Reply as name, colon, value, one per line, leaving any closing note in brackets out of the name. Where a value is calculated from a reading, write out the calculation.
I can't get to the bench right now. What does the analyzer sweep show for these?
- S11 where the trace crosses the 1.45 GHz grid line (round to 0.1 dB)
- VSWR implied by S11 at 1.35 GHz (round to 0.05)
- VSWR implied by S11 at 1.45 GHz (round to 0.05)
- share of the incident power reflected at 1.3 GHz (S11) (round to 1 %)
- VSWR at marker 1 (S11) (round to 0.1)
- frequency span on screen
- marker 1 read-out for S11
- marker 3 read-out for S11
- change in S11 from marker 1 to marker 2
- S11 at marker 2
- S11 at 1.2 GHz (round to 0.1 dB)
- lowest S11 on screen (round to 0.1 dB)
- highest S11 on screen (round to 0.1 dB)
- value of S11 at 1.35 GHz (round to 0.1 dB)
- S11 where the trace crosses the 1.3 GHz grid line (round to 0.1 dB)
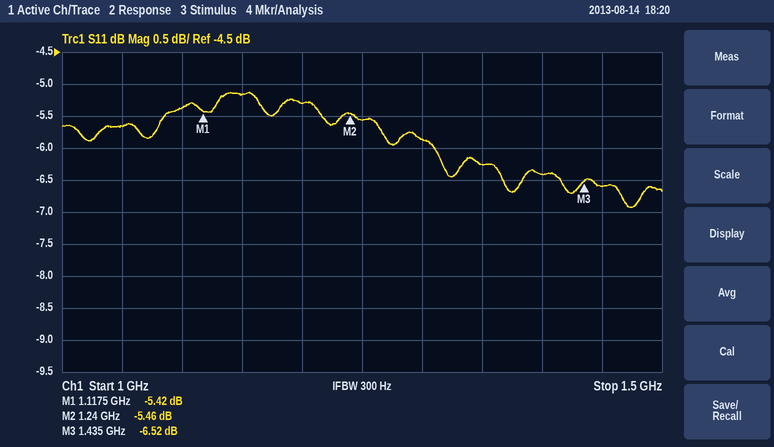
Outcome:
S11 where the trace crosses the 1.45 GHz grid line: -6.6 dB
VSWR implied by S11 at 1.35 GHz: |Γ| = 10^(-6.3/20) = 0.4842; VSWR = (1 + 0.4842)/(1 − 0.4842) ≈ 2.88, so 2.90 to the nearest 0.05
VSWR implied by S11 at 1.45 GHz: |Γ| = 10^(-6.6/20) = 0.4677; VSWR = (1 + 0.4677)/(1 − 0.4677) ≈ 2.76, so 2.75 to the nearest 0.05
share of the incident power reflected at 1.3 GHz (S11): 10^(-5.9/10) ≈ 26 %
VSWR at marker 1 (S11): (1 + 0.5358)/(1 − 0.5358) ≈ 3.3
frequency span on screen: 500 MHz
marker 1 read-out for S11: -5.42 dB
marker 3 read-out for S11: -6.52 dB
change in S11 from marker 1 to marker 2: -5.46 − (-5.42) = -0.04 dB
S11 at marker 2: -5.46 dB
S11 at 1.2 GHz: -5.3 dB
lowest S11 on screen: -6.9 dB
highest S11 on screen: -5.1 dB
value of S11 at 1.35 GHz: -6.3 dB
S11 where the trace crosses the 1.3 GHz grid line: -5.9 dB
